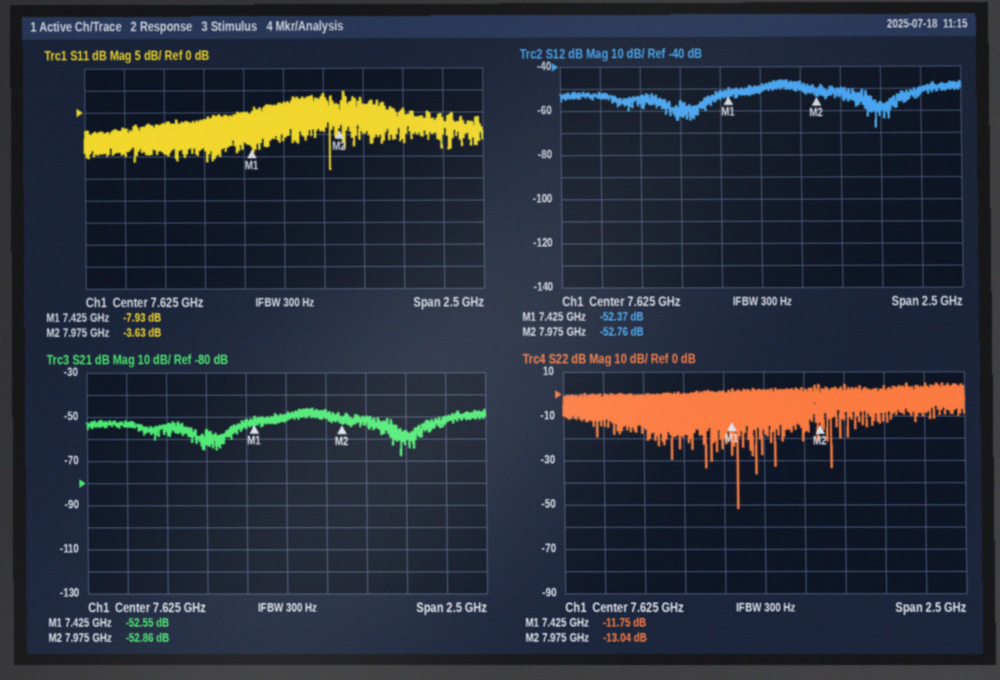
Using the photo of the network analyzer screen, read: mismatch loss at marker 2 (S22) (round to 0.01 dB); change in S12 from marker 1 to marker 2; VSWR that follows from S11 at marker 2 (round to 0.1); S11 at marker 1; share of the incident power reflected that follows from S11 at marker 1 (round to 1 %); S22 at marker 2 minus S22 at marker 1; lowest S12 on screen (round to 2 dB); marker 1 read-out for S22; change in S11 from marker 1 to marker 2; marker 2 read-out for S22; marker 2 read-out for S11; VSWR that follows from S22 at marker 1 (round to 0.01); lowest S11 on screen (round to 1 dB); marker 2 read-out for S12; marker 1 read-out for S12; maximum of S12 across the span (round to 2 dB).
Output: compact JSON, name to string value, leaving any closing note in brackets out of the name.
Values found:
{"mismatch loss at marker 2 (S22)": "0.22 dB", "change in S12 from marker 1 to marker 2": "-0.39 dB", "VSWR that follows from S11 at marker 2": "4.9", "S11 at marker 1": "-7.93 dB", "share of the incident power reflected that follows from S11 at marker 1": "16 %", "S22 at marker 2 minus S22 at marker 1": "-1.29 dB", "lowest S12 on screen": "-68 dB", "marker 1 read-out for S22": "-11.75 dB", "change in S11 from marker 1 to marker 2": "4.30 dB", "marker 2 read-out for S22": "-13.04 dB", "marker 2 read-out for S11": "-3.63 dB", "VSWR that follows from S22 at marker 1": "1.70", "lowest S11 on screen": "-13 dB", "marker 2 read-out for S12": "-52.76 dB", "marker 1 read-out for S12": "-52.37 dB", "maximum of S12 across the span": "-46 dB"}
